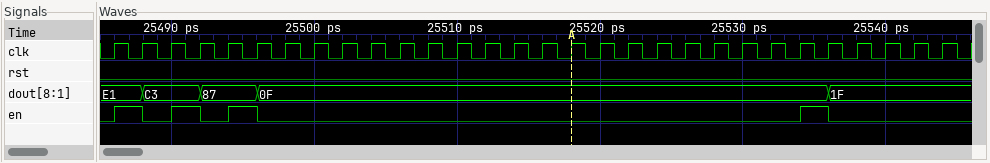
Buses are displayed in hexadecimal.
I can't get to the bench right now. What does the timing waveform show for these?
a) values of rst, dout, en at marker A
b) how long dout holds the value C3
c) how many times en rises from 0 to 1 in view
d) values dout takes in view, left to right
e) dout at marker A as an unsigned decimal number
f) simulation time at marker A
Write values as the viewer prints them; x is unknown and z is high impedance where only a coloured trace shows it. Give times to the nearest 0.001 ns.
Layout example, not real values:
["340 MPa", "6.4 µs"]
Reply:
["rst=0, dout=0F, en=0", "0.004 ns", "4", "E1, C3, 87, 0F, 1F", "15", "25.518 ns"]
